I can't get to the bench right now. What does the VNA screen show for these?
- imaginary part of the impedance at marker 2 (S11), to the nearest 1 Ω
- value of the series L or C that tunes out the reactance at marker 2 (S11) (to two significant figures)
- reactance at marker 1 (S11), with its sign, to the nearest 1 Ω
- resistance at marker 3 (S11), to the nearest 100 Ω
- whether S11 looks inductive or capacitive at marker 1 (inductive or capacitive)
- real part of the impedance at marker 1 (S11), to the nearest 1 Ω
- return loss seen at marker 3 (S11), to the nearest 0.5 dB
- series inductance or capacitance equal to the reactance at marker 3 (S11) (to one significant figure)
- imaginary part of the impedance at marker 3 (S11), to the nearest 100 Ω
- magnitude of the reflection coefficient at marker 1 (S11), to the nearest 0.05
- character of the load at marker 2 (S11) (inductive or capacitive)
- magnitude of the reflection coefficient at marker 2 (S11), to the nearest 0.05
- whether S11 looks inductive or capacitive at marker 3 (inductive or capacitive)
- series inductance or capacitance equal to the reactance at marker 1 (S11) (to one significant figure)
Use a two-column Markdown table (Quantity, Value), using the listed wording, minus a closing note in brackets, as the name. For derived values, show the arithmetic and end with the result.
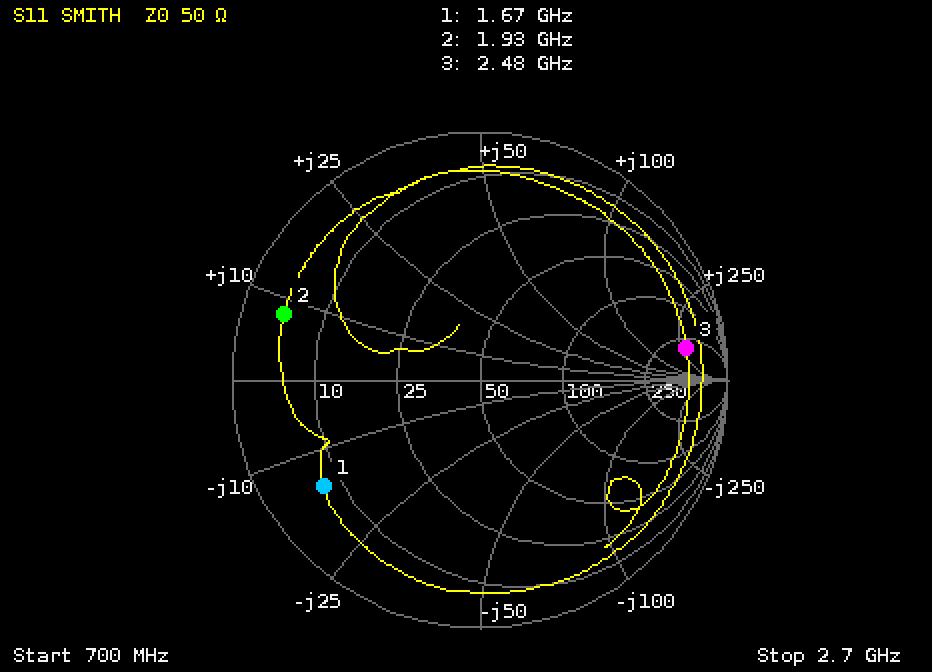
| Quantity | Value |
|---|---|
| imaginary part of the impedance at marker 2 (S11), to the nearest 1 Ω | +8 Ω |
| value of the series L or C that tunes out the reactance at marker 2 (S11) | C = 1/(2π × 1.93 GHz × 8 Ω) ≈ 10 pF |
| reactance at marker 1 (S11), with its sign, to the nearest 1 Ω | -15 Ω |
| resistance at marker 3 (S11), to the nearest 100 Ω | 300 Ω |
| whether S11 looks inductive or capacitive at marker 1 | capacitive |
| real part of the impedance at marker 1 (S11), to the nearest 1 Ω | 7 Ω |
| return loss seen at marker 3 (S11), to the nearest 0.5 dB | 1.5 dB |
| series inductance or capacitance equal to the reactance at marker 3 (S11) | L = 300 Ω/(2π × 2.48 GHz) ≈ 19.3 nH, so 20 nH to one significant figure |
| imaginary part of the impedance at marker 3 (S11), to the nearest 100 Ω | +300 Ω |
| magnitude of the reflection coefficient at marker 1 (S11), to the nearest 0.05 | 0.75 |
| character of the load at marker 2 (S11) | inductive |
| magnitude of the reflection coefficient at marker 2 (S11), to the nearest 0.05 | 0.85 |
| whether S11 looks inductive or capacitive at marker 3 | inductive |
| series inductance or capacitance equal to the reactance at marker 1 (S11) | C = 1/(2π × 1.67 GHz × 15 Ω) ≈ 6 pF |
